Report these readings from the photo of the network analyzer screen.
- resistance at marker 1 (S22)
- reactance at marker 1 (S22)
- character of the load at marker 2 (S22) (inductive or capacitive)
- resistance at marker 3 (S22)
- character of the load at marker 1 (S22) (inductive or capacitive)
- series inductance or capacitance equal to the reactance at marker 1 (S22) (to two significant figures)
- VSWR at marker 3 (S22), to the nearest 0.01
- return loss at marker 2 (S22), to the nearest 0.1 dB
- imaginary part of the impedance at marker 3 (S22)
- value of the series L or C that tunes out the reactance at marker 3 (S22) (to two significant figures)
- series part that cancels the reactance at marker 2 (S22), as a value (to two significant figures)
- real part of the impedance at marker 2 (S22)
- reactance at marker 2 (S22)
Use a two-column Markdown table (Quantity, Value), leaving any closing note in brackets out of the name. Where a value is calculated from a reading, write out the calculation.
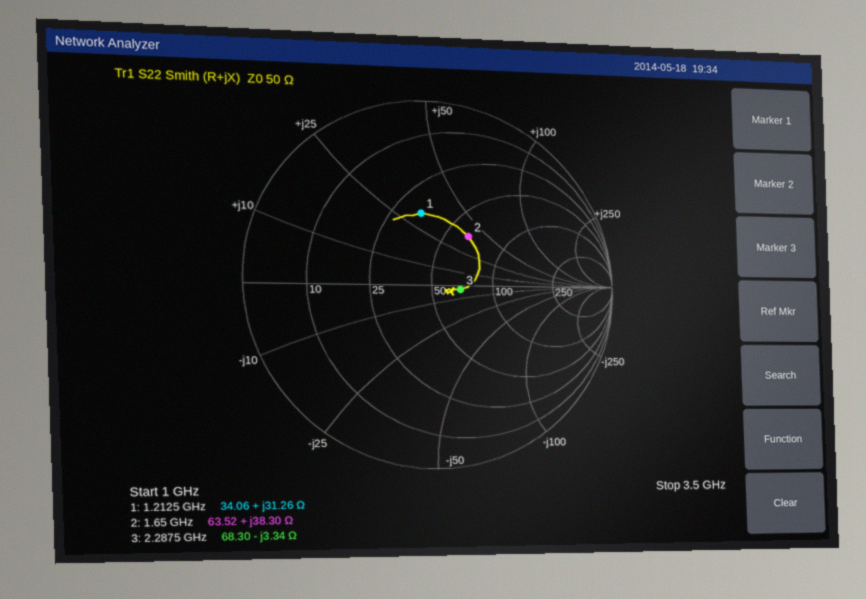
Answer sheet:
| Quantity | Value |
|---|---|
| resistance at marker 1 | 34.06 Ω |
| reactance at marker 1 | +31.26 Ω |
| character of the load at marker 2 (S22) | inductive |
| resistance at marker 3 | 68.30 Ω |
| character of the load at marker 1 (S22) | inductive |
| series inductance or capacitance equal to the reactance at marker 1 (S22) | L = 31.26 Ω/(2π × 1.2125 GHz) ≈ 4.1 nH |
| VSWR at marker 3 (S22), to the nearest 0.01 | 1.37 |
| return loss at marker 2 (S22), to the nearest 0.1 dB | 9.4 dB |
| imaginary part of the impedance at marker 3 | -3.34 Ω |
| value of the series L or C that tunes out the reactance at marker 3 (S22) | L = 3.34 Ω/(2π × 2.2875 GHz) ≈ 232 pH, so 230 pH to two significant figures |
| series part that cancels the reactance at marker 2 (S22), as a value | C = 1/(2π × 1.65 GHz × 38.3 Ω) ≈ 2.5 pF |
| real part of the impedance at marker 2 | 63.52 Ω |
| reactance at marker 2 | +38.30 Ω |
